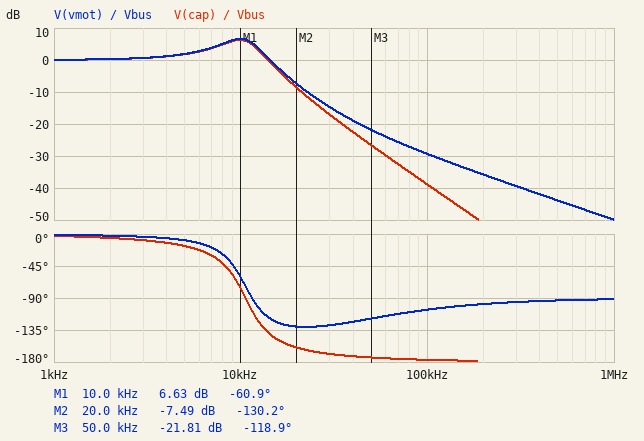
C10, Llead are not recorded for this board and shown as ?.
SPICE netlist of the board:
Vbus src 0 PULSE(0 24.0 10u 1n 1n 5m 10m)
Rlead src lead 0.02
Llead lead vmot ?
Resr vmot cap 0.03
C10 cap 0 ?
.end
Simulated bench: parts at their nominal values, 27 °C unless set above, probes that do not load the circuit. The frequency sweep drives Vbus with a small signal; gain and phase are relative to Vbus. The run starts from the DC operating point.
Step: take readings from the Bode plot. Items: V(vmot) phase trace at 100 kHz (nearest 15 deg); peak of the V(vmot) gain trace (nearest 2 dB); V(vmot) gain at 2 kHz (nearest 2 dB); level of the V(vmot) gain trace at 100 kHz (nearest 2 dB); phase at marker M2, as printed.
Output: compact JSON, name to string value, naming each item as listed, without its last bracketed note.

{"V(vmot) phase trace at 100 kHz": "-105 deg", "peak of the V(vmot) gain trace": "6 dB", "V(vmot) gain at 2 kHz": "0 dB", "level of the V(vmot) gain trace at 100 kHz": "-30 dB", "phase at marker M2, as printed": "-130.2 deg"}
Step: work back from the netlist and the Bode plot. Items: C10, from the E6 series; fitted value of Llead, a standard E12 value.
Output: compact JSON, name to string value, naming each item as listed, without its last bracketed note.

{"C10, from the E6 series": "150 µF", "fitted value of Llead, a standard E12 value": "1.5 µH"}
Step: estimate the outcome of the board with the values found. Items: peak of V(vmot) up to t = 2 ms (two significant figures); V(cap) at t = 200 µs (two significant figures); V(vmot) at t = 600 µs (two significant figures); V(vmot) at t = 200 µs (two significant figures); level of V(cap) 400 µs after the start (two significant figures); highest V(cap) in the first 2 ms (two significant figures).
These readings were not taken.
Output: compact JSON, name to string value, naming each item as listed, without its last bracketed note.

{"peak of V(vmot) up to t = 2 ms": "35 V", "V(cap) at t = 200 µs": "23 V", "V(vmot) at t = 600 µs": "24 V", "V(vmot) at t = 200 µs": "23 V", "level of V(cap) 400 µs after the start": "24 V", "highest V(cap) in the first 2 ms": "35 V"}
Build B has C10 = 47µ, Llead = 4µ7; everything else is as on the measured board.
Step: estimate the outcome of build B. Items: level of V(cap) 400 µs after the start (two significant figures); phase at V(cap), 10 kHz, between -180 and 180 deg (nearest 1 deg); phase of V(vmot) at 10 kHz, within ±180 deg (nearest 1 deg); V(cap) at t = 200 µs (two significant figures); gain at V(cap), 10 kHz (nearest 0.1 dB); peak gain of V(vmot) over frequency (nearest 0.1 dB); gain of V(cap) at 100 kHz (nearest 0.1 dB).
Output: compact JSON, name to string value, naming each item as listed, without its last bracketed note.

{"level of V(cap) 400 µs after the start": "22 V", "phase at V(cap), 10 kHz, between -180 and 180 deg": "-49 deg", "phase of V(vmot) at 10 kHz, within ±180 deg": "-44 deg", "V(cap) at t = 200 µs": "15 V", "gain at V(cap), 10 kHz": "14.2 dB", "peak gain of V(vmot) over frequency": "16.1 dB", "gain of V(cap) at 100 kHz": "-38.7 dB"}
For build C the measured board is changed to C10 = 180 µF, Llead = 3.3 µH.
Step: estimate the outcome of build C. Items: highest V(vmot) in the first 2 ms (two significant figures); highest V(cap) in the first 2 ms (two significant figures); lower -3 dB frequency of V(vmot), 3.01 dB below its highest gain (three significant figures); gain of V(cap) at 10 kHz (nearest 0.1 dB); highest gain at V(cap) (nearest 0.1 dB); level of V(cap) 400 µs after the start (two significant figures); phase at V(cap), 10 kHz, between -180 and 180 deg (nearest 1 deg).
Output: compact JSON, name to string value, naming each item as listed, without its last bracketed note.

{"highest V(vmot) in the first 2 ms": "38 V", "highest V(cap) in the first 2 ms": "37 V", "lower -3 dB frequency of V(vmot), 3.01 dB below its highest gain": "4.95 kHz", "gain of V(cap) at 10 kHz": "-3.3 dB", "highest gain at V(cap)": "8.8 dB", "level of V(cap) 400 µs after the start": "25 V", "phase at V(cap), 10 kHz, between -180 and 180 deg": "-157 deg"}
